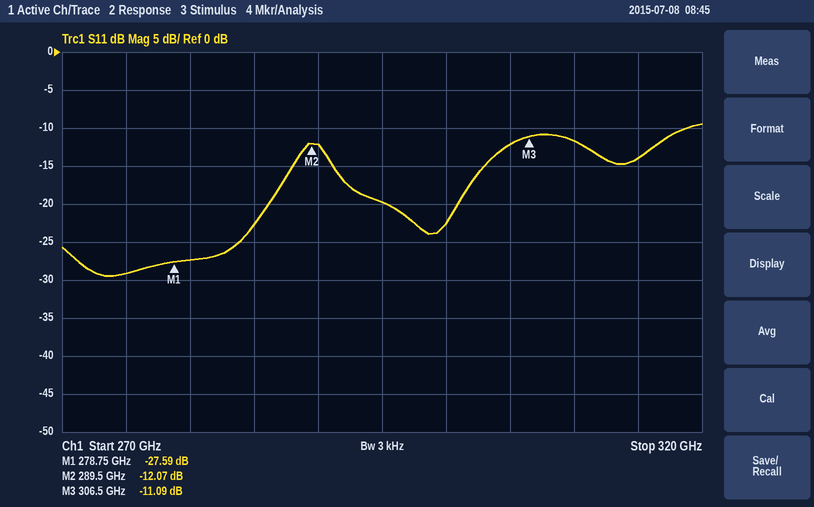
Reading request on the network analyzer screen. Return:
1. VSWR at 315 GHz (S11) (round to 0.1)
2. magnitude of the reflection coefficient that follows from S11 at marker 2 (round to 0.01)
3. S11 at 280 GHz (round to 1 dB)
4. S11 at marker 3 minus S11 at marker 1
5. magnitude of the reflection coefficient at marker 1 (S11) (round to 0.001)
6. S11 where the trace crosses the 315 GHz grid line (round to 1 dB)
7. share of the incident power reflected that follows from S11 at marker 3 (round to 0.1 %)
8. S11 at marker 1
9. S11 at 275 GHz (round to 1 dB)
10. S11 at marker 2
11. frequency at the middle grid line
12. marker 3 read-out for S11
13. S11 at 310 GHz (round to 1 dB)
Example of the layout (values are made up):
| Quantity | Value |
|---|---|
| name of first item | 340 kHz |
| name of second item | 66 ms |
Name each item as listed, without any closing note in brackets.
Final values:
| Quantity | Value |
|---|---|
| VSWR at 315 GHz (S11) | 1.5 |
| magnitude of the reflection coefficient that follows from S11 at marker 2 | 0.25 |
| S11 at 280 GHz | -27 dB |
| S11 at marker 3 minus S11 at marker 1 | 16.50 dB |
| magnitude of the reflection coefficient at marker 1 (S11) | 0.042 |
| S11 where the trace crosses the 315 GHz grid line | -14 dB |
| share of the incident power reflected that follows from S11 at marker 3 | 7.8 % |
| S11 at marker 1 | -27.59 dB |
| S11 at 275 GHz | -29 dB |
| S11 at marker 2 | -12.07 dB |
| frequency at the middle grid line | 295 GHz |
| marker 3 read-out for S11 | -11.09 dB |
| S11 at 310 GHz | -12 dB |
